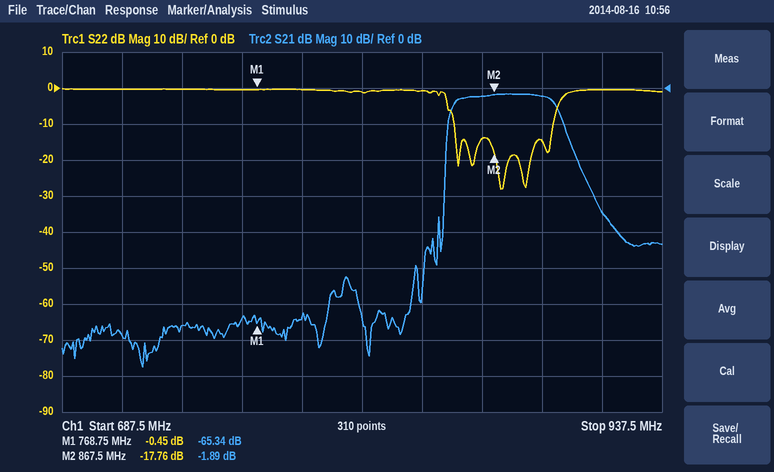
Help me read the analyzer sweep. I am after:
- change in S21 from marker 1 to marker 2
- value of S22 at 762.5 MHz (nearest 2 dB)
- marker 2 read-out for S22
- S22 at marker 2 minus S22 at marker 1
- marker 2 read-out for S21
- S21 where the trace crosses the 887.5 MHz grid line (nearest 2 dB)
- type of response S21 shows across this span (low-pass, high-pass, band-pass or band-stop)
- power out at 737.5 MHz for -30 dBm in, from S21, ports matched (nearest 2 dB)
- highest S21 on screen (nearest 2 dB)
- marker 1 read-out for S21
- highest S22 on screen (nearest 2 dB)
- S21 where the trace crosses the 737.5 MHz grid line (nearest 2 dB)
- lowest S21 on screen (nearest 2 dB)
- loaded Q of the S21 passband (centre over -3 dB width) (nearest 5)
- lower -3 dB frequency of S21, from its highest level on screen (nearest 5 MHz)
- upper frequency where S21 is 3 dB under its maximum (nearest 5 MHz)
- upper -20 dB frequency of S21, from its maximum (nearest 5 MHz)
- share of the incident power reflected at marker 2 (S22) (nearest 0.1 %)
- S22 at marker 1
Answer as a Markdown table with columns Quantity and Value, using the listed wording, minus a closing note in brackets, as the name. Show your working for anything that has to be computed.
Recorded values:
| Quantity | Value |
|---|---|
| change in S21 from marker 1 to marker 2 | -1.89 − (-65.34) = 63.45 dB |
| value of S22 at 762.5 MHz | 0 dB |
| marker 2 read-out for S22 | -17.76 dB |
| S22 at marker 2 minus S22 at marker 1 | -17.76 − (-0.45) = -17.31 dB |
| marker 2 read-out for S21 | -1.89 dB |
| S21 where the trace crosses the 887.5 MHz grid line | -2 dB |
| type of response S21 shows across this span | band-pass |
| power out at 737.5 MHz for -30 dBm in, from S21, ports matched | -30 dBm + (-66 dB) = -96 dBm |
| highest S21 on screen | -2 dB |
| marker 1 read-out for S21 | -65.34 dB |
| highest S22 on screen | 0 dB |
| S21 where the trace crosses the 737.5 MHz grid line | -66 dB |
| lowest S21 on screen | -78 dB |
| loaded Q of the S21 passband (centre over -3 dB width) | 872.5 MHz / 45 MHz ≈ 19.4, so 20 to the nearest 5 |
| lower -3 dB frequency of S21, from its highest level on screen | 850 MHz |
| upper frequency where S21 is 3 dB under its maximum | 895 MHz |
| upper -20 dB frequency of S21, from its maximum | 905 MHz |
| share of the incident power reflected at marker 2 (S22) | 10^(-17.76/10) ≈ 1.7 % |
| S22 at marker 1 | -0.45 dB |
